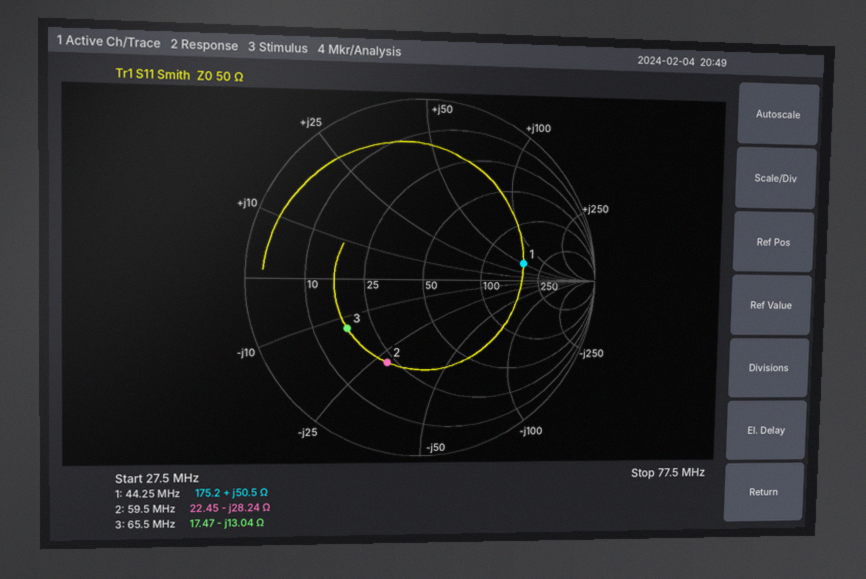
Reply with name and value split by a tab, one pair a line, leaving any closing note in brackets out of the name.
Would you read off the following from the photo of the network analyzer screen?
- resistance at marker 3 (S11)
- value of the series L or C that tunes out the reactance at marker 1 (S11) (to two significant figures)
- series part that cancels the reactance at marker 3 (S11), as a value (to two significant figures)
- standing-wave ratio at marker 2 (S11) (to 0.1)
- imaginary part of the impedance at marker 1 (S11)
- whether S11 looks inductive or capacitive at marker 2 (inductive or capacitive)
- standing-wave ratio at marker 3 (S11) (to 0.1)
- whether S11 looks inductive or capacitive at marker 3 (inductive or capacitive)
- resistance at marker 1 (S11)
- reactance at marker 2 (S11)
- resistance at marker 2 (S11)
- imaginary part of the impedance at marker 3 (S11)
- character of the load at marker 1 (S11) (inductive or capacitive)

resistance at marker 3	17.47 Ω
value of the series L or C that tunes out the reactance at marker 1 (S11)	71 pF
series part that cancels the reactance at marker 3 (S11), as a value	32 nH
standing-wave ratio at marker 2 (S11)	3.1
imaginary part of the impedance at marker 1	+50.5 Ω
whether S11 looks inductive or capacitive at marker 2	capacitive
standing-wave ratio at marker 3 (S11)	3.1
whether S11 looks inductive or capacitive at marker 3	capacitive
resistance at marker 1	175.2 Ω
reactance at marker 2	-28.24 Ω
resistance at marker 2	22.45 Ω
imaginary part of the impedance at marker 3	-13.04 Ω
character of the load at marker 1 (S11)	inductive
